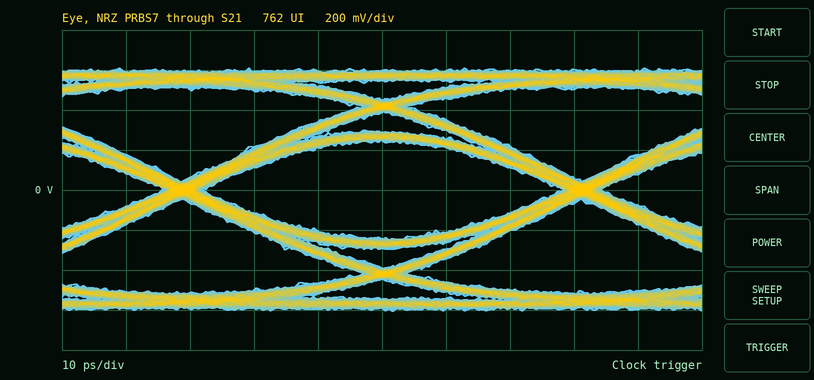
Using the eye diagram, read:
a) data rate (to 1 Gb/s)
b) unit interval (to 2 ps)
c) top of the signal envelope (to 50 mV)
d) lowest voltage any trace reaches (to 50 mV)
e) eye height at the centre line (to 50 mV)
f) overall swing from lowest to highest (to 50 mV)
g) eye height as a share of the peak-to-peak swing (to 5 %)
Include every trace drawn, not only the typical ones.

16 Gb/s
62 ps
600 mV
-600 mV
500 mV
1.20 V
40 %
